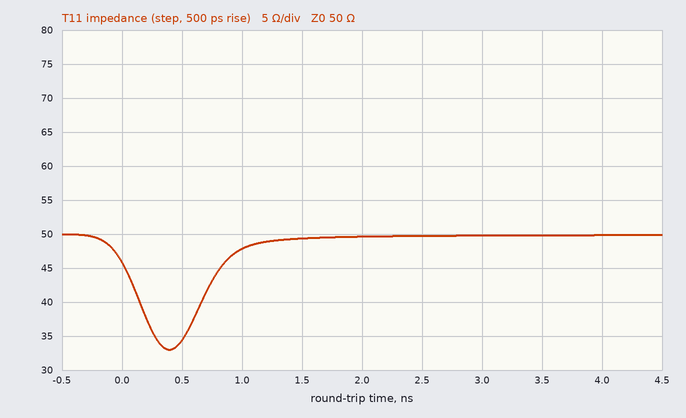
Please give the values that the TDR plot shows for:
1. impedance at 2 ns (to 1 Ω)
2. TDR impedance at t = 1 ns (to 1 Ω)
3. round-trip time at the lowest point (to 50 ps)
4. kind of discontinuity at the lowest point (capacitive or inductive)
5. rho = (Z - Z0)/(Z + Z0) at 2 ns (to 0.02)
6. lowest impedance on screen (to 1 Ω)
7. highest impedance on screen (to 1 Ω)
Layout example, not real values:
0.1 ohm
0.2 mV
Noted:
50 Ω
48 Ω
400 ps
capacitive
0.00
33 Ω
50 Ω
